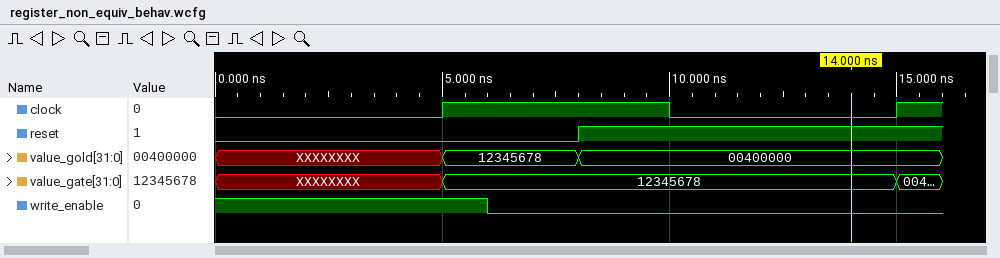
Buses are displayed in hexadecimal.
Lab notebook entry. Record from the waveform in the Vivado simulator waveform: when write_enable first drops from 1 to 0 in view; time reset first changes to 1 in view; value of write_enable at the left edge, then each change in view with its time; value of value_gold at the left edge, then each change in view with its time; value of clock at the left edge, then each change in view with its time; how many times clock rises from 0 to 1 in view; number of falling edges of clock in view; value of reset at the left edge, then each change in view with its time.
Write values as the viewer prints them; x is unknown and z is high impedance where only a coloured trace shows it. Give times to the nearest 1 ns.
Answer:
6 ns
8 ns
1, 0 at 6 ns
XXXXXXXX, 12345678 at 5 ns, 00400000 at 8 ns
0, 1 at 5 ns, 0 at 10 ns, 1 at 15 ns
2
1
0, 1 at 8 ns
